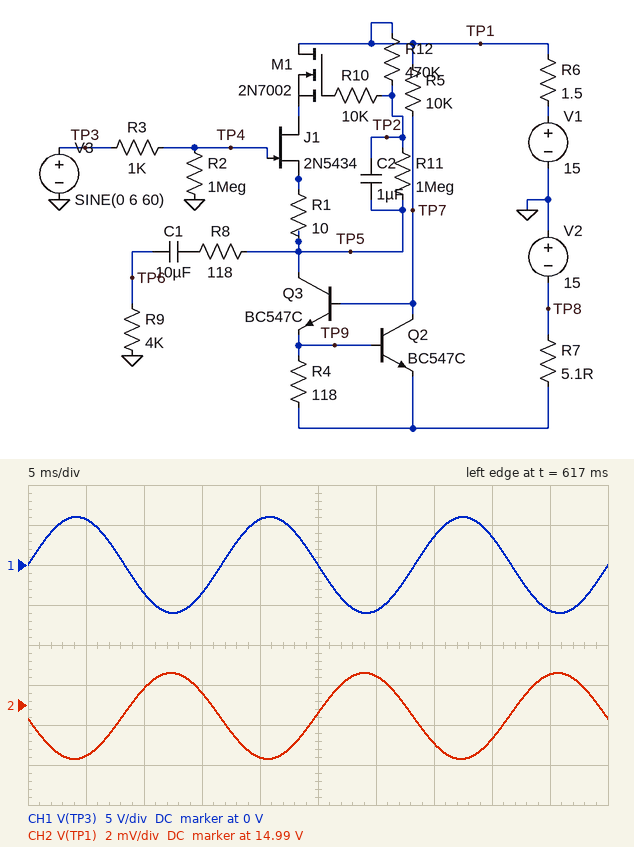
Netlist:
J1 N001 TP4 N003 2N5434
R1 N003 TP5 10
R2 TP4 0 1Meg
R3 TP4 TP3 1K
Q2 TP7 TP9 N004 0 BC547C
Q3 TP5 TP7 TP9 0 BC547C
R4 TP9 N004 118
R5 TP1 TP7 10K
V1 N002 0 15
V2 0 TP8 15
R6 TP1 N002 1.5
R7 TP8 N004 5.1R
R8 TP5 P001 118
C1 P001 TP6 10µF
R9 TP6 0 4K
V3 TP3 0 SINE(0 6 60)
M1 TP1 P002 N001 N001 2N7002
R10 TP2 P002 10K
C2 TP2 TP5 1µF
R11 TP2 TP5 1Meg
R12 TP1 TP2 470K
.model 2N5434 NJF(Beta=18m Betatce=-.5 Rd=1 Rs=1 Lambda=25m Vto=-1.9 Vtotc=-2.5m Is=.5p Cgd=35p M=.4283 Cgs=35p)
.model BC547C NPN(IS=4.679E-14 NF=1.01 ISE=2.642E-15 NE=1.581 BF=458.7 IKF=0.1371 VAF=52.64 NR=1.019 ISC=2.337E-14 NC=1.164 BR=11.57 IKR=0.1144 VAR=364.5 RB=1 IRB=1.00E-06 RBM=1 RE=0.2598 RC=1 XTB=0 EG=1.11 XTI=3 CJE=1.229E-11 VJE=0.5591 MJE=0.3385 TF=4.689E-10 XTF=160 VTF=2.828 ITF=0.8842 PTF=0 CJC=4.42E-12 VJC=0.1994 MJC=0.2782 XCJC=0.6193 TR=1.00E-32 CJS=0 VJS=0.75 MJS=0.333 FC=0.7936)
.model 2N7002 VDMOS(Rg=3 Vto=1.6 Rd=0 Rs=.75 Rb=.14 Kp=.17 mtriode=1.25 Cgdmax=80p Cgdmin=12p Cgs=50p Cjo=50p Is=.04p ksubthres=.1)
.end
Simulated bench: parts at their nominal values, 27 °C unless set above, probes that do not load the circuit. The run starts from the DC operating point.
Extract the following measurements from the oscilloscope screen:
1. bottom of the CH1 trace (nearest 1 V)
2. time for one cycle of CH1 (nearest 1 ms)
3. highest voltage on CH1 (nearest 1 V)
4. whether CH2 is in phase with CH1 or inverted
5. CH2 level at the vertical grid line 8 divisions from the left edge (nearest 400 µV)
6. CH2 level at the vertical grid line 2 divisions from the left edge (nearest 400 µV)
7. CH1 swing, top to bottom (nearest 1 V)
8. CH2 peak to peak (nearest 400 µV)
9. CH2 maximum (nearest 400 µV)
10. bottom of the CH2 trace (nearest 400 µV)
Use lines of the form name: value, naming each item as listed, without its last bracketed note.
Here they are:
bottom of the CH1 trace: -6 V
time for one cycle of CH1: 17 ms
highest voltage on CH1: 6 V
whether CH2 is in phase with CH1 or inverted: inverted
CH2 level at the vertical grid line 8 divisions from the left edge: 14.9864 V
CH2 level at the vertical grid line 2 divisions from the left edge: 14.9888 V
CH1 swing, top to bottom: 12 V
CH2 peak to peak: 4.4 mV
CH2 maximum: 14.9896 V
bottom of the CH2 trace: 14.9852 V
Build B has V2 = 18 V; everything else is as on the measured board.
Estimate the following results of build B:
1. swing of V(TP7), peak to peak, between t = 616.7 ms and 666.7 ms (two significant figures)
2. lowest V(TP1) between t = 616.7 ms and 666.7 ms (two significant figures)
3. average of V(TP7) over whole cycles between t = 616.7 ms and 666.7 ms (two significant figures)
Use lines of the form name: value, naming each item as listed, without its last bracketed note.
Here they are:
swing of V(TP7), peak to peak, between t = 616.7 ms and 666.7 ms: 4.5 mV
lowest V(TP1) between t = 616.7 ms and 666.7 ms: 15 V
average of V(TP7) over whole cycles between t = 616.7 ms and 666.7 ms: -17 V
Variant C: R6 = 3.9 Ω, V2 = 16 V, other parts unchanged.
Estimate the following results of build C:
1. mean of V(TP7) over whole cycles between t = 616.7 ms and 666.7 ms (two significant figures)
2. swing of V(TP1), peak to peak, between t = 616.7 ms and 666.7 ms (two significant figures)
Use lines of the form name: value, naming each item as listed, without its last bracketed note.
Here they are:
mean of V(TP7) over whole cycles between t = 616.7 ms and 666.7 ms: -15 V
swing of V(TP1), peak to peak, between t = 616.7 ms and 666.7 ms: 11 mV
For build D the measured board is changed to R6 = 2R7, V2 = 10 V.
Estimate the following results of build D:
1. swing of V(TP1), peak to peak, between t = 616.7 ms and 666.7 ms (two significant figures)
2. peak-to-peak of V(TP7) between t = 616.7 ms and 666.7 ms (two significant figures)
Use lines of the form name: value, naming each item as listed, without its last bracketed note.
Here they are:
swing of V(TP1), peak to peak, between t = 616.7 ms and 666.7 ms: 7.7 mV
peak-to-peak of V(TP7) between t = 616.7 ms and 666.7 ms: 5.1 mV
